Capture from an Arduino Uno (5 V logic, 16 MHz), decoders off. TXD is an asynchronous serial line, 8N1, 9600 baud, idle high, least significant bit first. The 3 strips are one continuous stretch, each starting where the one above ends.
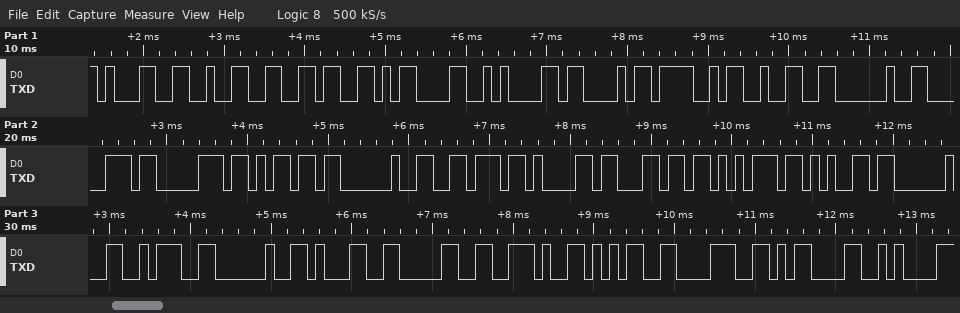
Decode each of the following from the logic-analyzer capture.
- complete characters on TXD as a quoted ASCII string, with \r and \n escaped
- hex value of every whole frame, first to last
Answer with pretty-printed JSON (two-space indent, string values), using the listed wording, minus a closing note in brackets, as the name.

{
  "complete characters on TXD as a quoted ASCII string, with \\r and \\n escaped": "\"126\\r\\nCO2 ppm value : 10.58\\r\\n\"",
  "hex value of every whole frame, first to last": "31 32 36 0D 0A 43 4F 32 20 70 70 6D 20 76 61 6C 75 65 20 3A 20 31 30 2E 35 38 0D 0A"
}
